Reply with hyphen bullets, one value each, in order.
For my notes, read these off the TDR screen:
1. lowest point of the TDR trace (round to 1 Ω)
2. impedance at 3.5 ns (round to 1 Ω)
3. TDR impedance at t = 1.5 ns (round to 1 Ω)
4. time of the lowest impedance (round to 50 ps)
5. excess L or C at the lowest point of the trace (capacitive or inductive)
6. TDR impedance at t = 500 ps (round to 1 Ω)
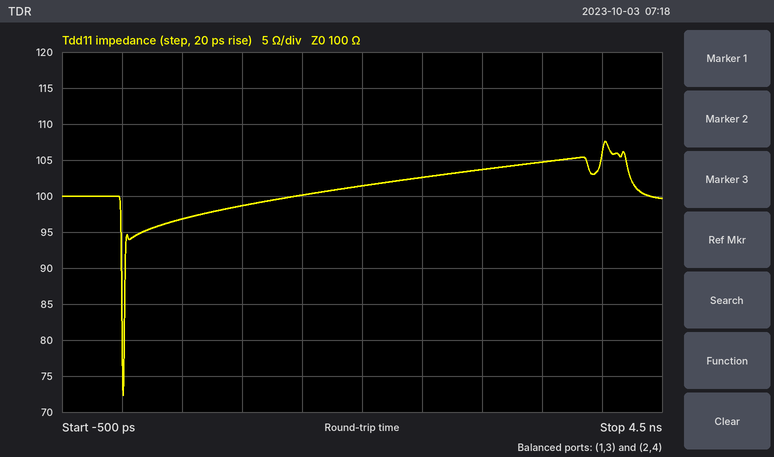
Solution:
- 72 Ω
- 105 Ω
- 100 Ω
- 0 ps
- capacitive
- 97 Ω
